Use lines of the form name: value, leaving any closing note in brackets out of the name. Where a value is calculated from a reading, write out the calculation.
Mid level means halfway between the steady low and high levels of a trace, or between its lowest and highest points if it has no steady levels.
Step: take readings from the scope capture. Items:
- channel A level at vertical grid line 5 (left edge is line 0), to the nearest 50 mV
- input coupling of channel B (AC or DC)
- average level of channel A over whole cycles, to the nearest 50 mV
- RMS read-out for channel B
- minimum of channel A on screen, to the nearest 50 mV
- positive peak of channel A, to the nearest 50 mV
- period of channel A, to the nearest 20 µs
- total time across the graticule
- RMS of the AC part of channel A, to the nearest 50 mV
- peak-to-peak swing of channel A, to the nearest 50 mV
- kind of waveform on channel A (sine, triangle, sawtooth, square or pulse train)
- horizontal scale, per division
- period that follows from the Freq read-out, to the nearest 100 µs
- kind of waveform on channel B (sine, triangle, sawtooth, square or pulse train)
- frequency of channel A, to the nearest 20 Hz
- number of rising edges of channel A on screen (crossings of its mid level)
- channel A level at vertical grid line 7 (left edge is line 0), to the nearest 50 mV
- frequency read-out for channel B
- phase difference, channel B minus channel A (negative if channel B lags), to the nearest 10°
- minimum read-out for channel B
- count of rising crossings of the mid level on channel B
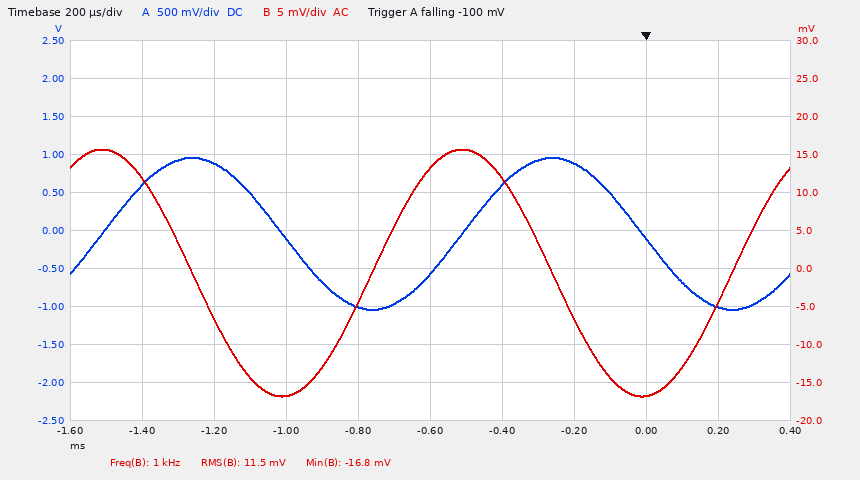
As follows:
channel A level at vertical grid line 5 (left edge is line 0), to the nearest 50 mV: -550 mV
input coupling of channel B: AC
average level of channel A over whole cycles, to the nearest 50 mV: (950 mV + (-1.05 V)) / 2 ≈ -50 mV
RMS read-out for channel B: 11.5 mV
minimum of channel A on screen, to the nearest 50 mV: -1.05 V
positive peak of channel A, to the nearest 50 mV: 950 mV
period of channel A, to the nearest 20 µs: 1.00 ms
total time across the graticule: 2 ms
RMS of the AC part of channel A, to the nearest 50 mV: 2.00 V / (2√2) ≈ 707 mV, so 700 mV to the nearest 50 mV
peak-to-peak swing of channel A, to the nearest 50 mV: 950 mV − (-1.05 V) = 2.00 V
kind of waveform on channel A: sine
horizontal scale, per division: 200 µs
period that follows from the Freq read-out, to the nearest 100 µs: 1 / 1 kHz ≈ 1.0 ms
kind of waveform on channel B: sine
frequency of channel A, to the nearest 20 Hz: 1 / 1.00 ms ≈ 1.00 kHz
number of rising edges of channel A on screen: 2
channel A level at vertical grid line 7 (left edge is line 0), to the nearest 50 mV: 900 mV
frequency read-out for channel B: 1 kHz
phase difference, channel B minus channel A (negative if channel B lags), to the nearest 10°: +90°
minimum read-out for channel B: -16.8 mV
count of rising crossings of the mid level on channel B: 2
